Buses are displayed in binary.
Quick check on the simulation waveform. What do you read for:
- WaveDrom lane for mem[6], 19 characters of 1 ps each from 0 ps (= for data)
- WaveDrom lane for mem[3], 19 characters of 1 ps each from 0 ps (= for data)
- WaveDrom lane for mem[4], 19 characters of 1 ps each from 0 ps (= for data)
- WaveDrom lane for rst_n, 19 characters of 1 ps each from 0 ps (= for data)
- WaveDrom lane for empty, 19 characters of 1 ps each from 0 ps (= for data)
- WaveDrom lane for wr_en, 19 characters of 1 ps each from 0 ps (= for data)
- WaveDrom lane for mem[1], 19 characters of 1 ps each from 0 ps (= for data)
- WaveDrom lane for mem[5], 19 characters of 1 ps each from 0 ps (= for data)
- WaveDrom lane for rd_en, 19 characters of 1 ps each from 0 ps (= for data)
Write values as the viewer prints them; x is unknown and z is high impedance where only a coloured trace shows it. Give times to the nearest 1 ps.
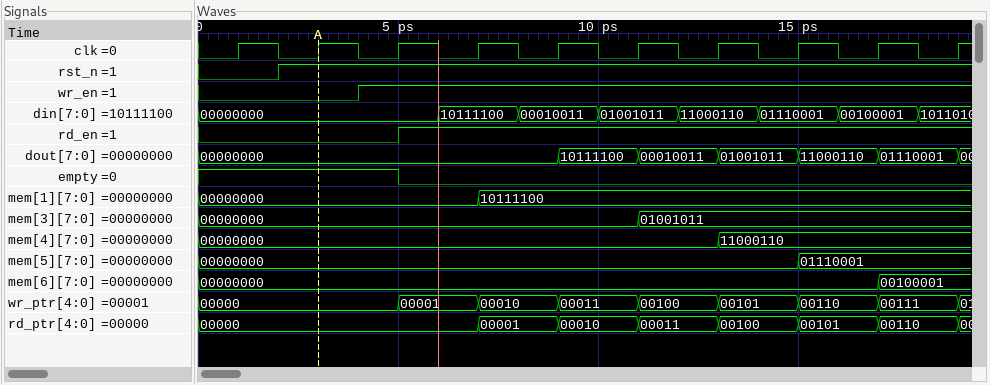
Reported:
{name: 'mem[6]', wave: '=................=.', data: '00000000 00100001'}
{name: 'mem[3]', wave: '=..........=.......', data: '00000000 01001011'}
{name: 'mem[4]', wave: '=............=.....', data: '00000000 11000110'}
{name: 'rst_n', wave: '0.1................'}
{name: 'empty', wave: '1....0.............'}
{name: 'wr_en', wave: '0...1..............'}
{name: 'mem[1]', wave: '=......=...........', data: '00000000 10111100'}
{name: 'mem[5]', wave: '=..............=...', data: '00000000 01110001'}
{name: 'rd_en', wave: '0....1.............'}
